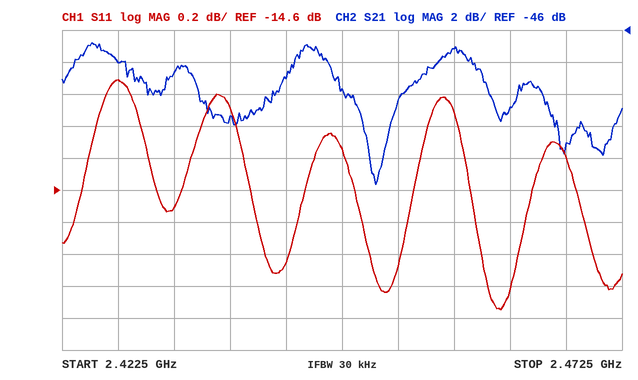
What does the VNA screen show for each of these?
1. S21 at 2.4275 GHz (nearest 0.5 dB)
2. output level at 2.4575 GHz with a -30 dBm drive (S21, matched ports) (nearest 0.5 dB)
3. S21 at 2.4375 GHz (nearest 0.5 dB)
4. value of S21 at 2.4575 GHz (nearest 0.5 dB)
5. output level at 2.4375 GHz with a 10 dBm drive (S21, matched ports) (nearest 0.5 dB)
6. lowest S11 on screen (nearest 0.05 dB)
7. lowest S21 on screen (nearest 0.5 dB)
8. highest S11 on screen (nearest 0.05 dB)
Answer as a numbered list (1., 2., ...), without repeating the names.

1. -48.0 dB
2. -77.0 dBm
3. -51.5 dB
4. -47.0 dB
5. -41.5 dBm
6. -15.35 dB
7. -55.5 dB
8. -13.90 dB
